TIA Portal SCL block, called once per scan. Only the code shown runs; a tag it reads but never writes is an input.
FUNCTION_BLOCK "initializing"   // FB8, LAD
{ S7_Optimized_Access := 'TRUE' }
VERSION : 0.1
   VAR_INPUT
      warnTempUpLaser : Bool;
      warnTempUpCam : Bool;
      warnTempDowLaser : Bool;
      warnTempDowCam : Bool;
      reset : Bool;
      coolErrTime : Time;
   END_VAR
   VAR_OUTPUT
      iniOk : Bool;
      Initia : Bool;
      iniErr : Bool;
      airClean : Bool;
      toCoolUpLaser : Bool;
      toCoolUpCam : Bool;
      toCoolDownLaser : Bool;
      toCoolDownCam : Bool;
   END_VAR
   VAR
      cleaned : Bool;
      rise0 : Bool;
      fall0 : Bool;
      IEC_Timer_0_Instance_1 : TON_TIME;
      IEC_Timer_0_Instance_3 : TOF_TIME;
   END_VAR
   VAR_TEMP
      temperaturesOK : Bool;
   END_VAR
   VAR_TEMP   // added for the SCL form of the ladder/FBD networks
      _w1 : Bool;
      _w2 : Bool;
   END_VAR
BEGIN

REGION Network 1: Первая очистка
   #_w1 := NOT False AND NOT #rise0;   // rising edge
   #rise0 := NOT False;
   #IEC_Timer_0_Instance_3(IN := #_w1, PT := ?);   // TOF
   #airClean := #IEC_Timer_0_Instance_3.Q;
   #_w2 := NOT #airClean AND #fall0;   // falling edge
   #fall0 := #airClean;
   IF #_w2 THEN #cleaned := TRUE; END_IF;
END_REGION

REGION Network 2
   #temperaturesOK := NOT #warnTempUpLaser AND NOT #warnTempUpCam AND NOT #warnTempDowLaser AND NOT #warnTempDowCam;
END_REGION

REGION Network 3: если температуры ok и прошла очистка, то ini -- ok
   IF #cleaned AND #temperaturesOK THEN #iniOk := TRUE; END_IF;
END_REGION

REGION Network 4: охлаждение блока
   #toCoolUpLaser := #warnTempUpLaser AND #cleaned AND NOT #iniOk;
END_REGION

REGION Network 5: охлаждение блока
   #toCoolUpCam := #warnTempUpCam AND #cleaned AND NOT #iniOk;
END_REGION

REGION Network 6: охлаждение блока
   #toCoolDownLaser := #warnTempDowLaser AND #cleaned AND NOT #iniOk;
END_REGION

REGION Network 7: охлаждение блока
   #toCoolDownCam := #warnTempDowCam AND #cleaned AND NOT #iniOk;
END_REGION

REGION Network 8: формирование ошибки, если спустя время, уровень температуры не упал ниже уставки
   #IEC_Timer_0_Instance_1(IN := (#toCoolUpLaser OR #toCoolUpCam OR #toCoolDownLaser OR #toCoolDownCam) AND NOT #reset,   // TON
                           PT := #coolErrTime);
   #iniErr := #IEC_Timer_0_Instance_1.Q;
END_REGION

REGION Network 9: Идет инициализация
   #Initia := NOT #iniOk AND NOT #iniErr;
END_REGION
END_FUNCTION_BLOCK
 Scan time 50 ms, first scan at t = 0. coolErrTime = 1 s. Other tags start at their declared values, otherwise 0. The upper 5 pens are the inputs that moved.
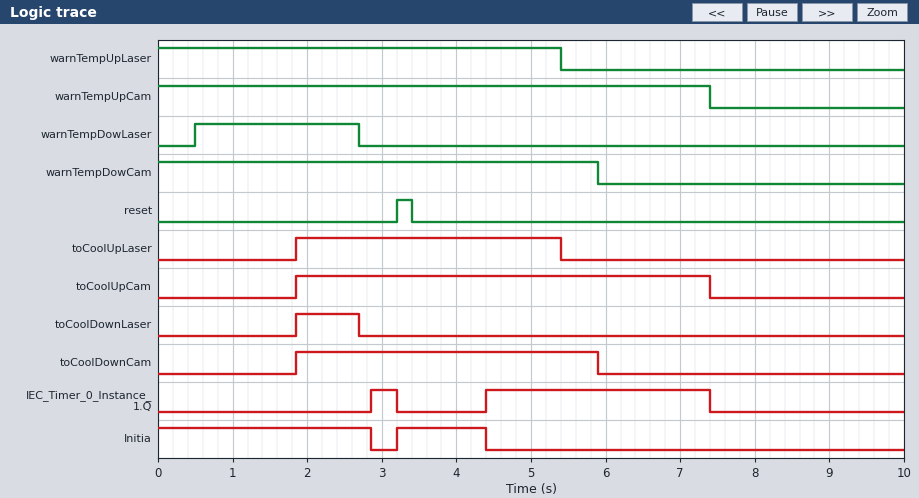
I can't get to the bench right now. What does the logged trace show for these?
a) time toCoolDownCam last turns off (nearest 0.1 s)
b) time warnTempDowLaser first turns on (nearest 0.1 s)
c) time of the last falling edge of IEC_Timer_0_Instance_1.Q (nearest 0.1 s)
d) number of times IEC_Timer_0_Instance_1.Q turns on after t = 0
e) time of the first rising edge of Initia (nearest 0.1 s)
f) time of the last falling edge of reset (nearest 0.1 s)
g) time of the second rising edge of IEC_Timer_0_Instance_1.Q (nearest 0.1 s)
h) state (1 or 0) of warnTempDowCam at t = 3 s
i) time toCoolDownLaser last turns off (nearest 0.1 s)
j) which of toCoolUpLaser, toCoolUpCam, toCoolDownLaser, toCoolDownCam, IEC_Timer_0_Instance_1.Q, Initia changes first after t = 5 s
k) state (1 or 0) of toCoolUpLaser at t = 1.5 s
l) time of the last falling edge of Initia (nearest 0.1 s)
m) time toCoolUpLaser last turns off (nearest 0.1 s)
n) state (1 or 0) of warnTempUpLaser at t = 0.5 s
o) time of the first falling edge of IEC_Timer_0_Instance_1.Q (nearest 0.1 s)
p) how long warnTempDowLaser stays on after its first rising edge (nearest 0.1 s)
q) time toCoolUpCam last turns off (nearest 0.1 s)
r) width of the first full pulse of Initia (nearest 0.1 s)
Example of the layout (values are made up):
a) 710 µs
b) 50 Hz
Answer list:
a) 5.9 s
b) 0.5 s
c) 7.4 s
d) 2
e) 3.2 s
f) 3.4 s
g) 4.4 s
h) 1
i) 2.7 s
j) toCoolUpLaser
k) 0
l) 4.4 s
m) 5.4 s
n) 1
o) 3.2 s
p) 2.2 s
q) 7.4 s
r) 1.2 s
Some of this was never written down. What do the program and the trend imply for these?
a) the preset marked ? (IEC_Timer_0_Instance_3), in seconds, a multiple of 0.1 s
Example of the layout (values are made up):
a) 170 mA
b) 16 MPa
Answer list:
a) 1.8 s
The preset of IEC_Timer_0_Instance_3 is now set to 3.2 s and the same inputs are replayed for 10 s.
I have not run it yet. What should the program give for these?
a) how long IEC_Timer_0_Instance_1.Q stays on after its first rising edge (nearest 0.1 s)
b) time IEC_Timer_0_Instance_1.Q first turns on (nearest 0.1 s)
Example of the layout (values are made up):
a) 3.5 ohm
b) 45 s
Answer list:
a) 3.0 s
b) 4.4 s
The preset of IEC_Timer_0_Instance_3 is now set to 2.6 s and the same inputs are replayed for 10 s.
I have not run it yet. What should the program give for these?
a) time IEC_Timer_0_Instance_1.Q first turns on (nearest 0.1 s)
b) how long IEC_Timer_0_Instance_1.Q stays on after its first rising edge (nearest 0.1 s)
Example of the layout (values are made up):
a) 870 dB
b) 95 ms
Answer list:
a) 4.4 s
b) 3.0 s
